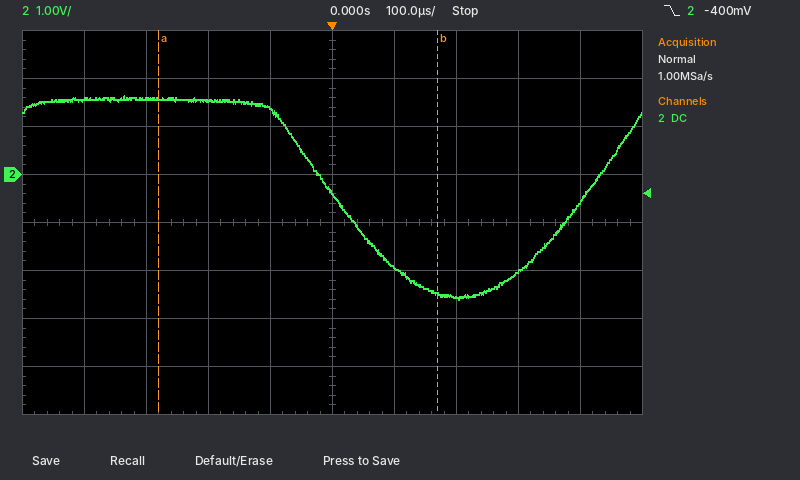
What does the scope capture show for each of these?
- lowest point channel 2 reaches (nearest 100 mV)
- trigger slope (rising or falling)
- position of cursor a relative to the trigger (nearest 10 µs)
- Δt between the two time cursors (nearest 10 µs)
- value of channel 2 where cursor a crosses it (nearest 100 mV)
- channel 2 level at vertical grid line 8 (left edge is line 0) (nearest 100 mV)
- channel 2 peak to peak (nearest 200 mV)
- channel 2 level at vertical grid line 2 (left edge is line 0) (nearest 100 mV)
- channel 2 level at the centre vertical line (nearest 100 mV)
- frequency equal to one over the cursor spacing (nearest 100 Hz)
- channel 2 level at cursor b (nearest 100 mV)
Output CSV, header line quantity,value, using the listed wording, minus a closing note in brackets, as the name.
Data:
quantity,value
lowest point channel 2 reaches,-2.6 V
trigger slope,falling
position of cursor a relative to the trigger,-280 µs
Δt between the two time cursors,450 µs
value of channel 2 where cursor a crosses it,1.6 V
channel 2 level at vertical grid line 8 (left edge is line 0),-2.0 V
channel 2 peak to peak,4.2 V
channel 2 level at vertical grid line 2 (left edge is line 0),1.6 V
channel 2 level at the centre vertical line,-400 mV
frequency equal to one over the cursor spacing,2.2 kHz
channel 2 level at cursor b,-2.5 V
